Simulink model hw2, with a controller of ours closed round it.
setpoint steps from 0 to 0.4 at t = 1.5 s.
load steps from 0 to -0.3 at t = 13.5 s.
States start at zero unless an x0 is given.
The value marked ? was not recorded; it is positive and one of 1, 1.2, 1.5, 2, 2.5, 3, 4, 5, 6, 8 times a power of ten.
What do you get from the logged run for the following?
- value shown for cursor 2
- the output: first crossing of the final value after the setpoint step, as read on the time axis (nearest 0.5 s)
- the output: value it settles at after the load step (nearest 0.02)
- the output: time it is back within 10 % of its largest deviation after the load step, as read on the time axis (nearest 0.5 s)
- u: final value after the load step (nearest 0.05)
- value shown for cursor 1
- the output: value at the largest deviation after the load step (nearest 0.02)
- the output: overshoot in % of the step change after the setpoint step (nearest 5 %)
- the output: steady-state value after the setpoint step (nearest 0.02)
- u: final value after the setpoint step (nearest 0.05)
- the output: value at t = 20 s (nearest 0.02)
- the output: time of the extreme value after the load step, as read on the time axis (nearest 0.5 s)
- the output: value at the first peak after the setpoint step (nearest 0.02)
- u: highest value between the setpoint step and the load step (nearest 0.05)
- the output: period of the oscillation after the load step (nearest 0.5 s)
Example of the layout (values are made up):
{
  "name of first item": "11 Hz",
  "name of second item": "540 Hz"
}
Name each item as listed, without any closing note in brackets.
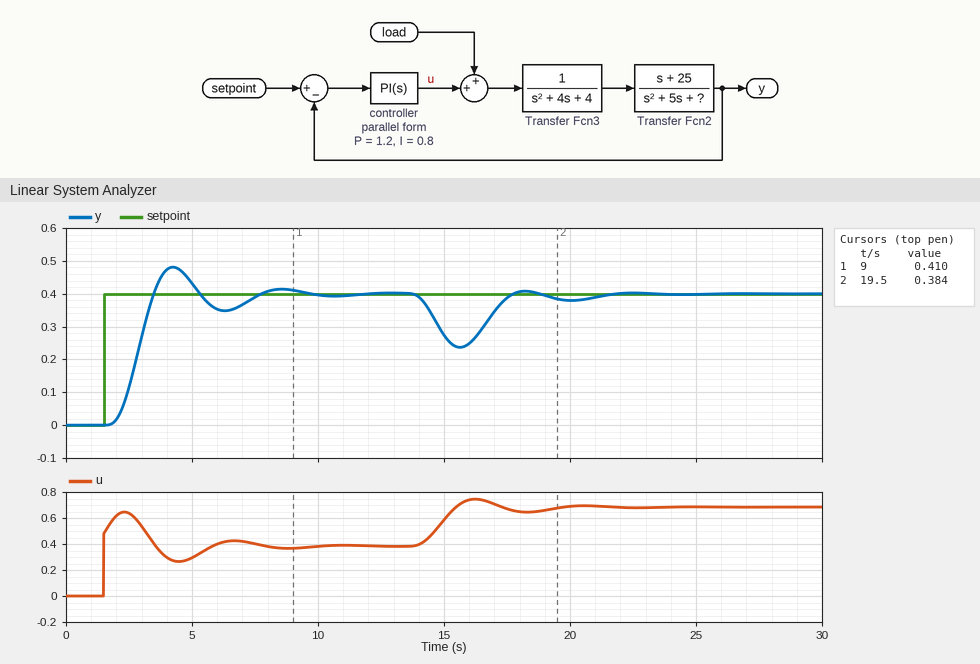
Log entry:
{
  "value shown for cursor 2": "0.384",
  "the output: first crossing of the final value after the setpoint step, as read on the time axis": "3.5 s",
  "the output: value it settles at after the load step": "0.40",
  "the output: time it is back within 10 % of its largest deviation after the load step, as read on the time axis": "20.5 s",
  "u: final value after the load step": "0.70",
  "value shown for cursor 1": "0.410",
  "the output: value at the largest deviation after the load step": "0.24",
  "the output: overshoot in % of the step change after the setpoint step": "20 %",
  "the output: steady-state value after the setpoint step": "0.40",
  "u: final value after the setpoint step": "0.40",
  "the output: value at t = 20 s": "0.38",
  "the output: time of the extreme value after the load step, as read on the time axis": "15.5 s",
  "the output: value at the first peak after the setpoint step": "0.48",
  "u: highest value between the setpoint step and the load step": "0.65",
  "the output: period of the oscillation after the load step": "4.5 s"
}
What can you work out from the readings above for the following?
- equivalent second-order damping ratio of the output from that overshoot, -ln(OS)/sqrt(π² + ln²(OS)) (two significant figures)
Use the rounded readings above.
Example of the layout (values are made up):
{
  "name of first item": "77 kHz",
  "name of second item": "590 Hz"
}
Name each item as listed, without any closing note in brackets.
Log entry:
{
  "equivalent second-order damping ratio of the output from that overshoot, -ln(OS)/sqrt(π² + ln²(OS))": "0.46"
}
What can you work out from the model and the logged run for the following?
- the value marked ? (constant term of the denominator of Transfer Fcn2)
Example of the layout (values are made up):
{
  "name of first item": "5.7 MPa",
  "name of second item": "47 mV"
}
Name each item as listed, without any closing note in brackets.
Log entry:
{
  "the value marked ?": "6"
}
